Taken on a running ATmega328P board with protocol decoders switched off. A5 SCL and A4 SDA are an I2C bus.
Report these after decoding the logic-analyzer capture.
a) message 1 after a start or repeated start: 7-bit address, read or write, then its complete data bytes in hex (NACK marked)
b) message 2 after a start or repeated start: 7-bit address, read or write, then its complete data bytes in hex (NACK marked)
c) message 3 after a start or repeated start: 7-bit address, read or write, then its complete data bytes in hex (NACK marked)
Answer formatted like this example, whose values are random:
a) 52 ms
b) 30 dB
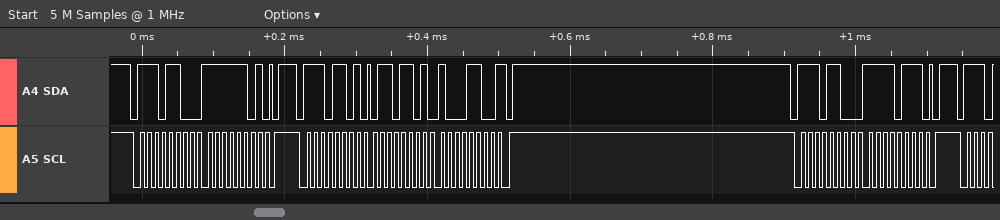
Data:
a) 0x76 write: FD
b) 0x76 read: 6D 8C NACK
c) 0x76 write: F7
